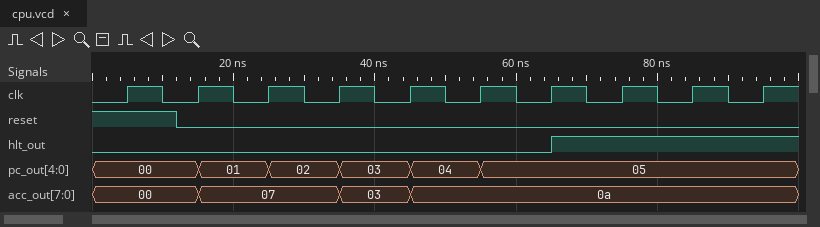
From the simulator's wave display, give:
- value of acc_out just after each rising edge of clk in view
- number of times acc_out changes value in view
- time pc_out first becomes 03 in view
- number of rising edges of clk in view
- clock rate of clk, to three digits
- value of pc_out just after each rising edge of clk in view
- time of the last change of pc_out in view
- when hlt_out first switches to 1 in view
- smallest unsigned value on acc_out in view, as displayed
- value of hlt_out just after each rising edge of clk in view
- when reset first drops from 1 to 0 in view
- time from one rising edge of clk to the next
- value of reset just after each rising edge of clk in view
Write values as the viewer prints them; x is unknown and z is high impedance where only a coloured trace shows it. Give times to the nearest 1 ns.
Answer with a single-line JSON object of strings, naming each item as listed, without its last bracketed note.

{"value of acc_out just after each rising edge of clk in view": "00, 07, 07, 03, 0a, 0a, 0a, 0a, 0a, 0a", "number of times acc_out changes value in view": "3", "time pc_out first becomes 03 in view": "35 ns", "number of rising edges of clk in view": "10", "clock rate of clk, to three digits": "100 MHz", "value of pc_out just after each rising edge of clk in view": "00, 01, 02, 03, 04, 05, 05, 05, 05, 05", "time of the last change of pc_out in view": "55 ns", "when hlt_out first switches to 1 in view": "65 ns", "smallest unsigned value on acc_out in view, as displayed": "00", "value of hlt_out just after each rising edge of clk in view": "0 0 0 0 0 0 1 1 1 1", "when reset first drops from 1 to 0 in view": "12 ns", "time from one rising edge of clk to the next": "10 ns", "value of reset just after each rising edge of clk in view": "1 0 0 0 0 0 0 0 0 0"}
